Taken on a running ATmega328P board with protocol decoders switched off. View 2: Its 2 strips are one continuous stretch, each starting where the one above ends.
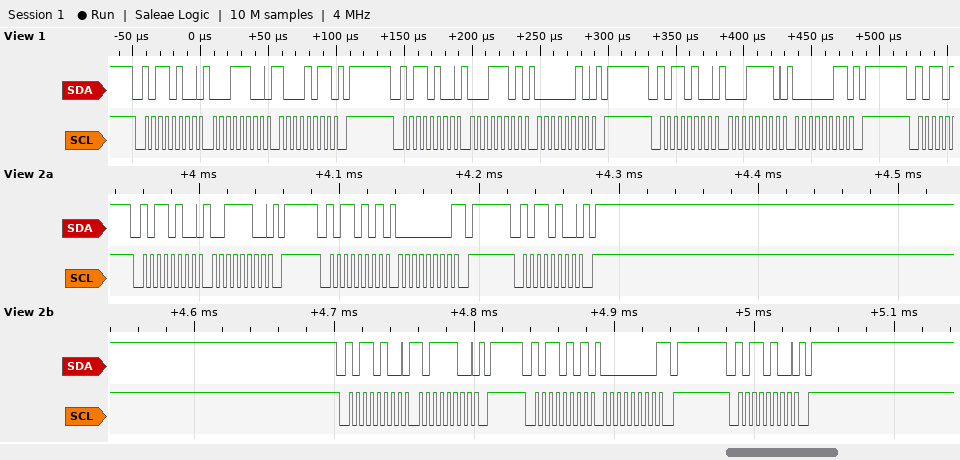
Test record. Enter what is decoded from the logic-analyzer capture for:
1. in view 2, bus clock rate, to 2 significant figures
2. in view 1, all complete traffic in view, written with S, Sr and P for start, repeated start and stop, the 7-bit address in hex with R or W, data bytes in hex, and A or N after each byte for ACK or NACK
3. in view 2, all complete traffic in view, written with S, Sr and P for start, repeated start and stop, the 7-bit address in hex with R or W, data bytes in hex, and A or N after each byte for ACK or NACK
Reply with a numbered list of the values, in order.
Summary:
1. 200 kHz
2. S 5AW A 1C A 8B A P S 5AW A 1D A 02 A P S 5AW A 1E A 03 A P
3. S 5AW A 3C A P S 5AR A 00 N P S 5AW A P S 5AW A BC A P S 5AR A 00 N P S 5AW A P
